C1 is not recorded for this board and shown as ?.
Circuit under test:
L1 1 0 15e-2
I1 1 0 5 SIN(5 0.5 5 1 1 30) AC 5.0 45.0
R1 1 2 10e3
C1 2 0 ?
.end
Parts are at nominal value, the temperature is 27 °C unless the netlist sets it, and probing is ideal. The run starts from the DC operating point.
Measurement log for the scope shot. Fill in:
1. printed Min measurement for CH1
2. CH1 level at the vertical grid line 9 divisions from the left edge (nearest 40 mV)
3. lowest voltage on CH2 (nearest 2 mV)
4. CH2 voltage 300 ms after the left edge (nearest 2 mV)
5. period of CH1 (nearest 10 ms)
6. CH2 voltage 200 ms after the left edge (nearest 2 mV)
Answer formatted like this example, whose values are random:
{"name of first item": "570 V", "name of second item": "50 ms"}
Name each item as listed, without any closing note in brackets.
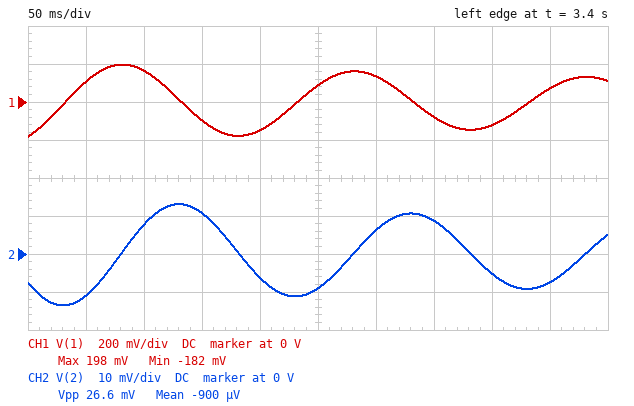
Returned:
{"printed Min measurement for CH1": "-182 mV", "CH1 level at the vertical grid line 9 divisions from the left edge": "80 mV", "lowest voltage on CH2": "-14 mV", "CH2 voltage 300 ms after the left edge": "6 mV", "period of CH1": "200 ms", "CH2 voltage 200 ms after the left edge": "-6 mV"}
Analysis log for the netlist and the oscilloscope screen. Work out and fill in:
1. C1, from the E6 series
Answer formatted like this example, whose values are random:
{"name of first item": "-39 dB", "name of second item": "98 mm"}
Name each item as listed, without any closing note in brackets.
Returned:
{"C1, from the E6 series": "47 µF"}
